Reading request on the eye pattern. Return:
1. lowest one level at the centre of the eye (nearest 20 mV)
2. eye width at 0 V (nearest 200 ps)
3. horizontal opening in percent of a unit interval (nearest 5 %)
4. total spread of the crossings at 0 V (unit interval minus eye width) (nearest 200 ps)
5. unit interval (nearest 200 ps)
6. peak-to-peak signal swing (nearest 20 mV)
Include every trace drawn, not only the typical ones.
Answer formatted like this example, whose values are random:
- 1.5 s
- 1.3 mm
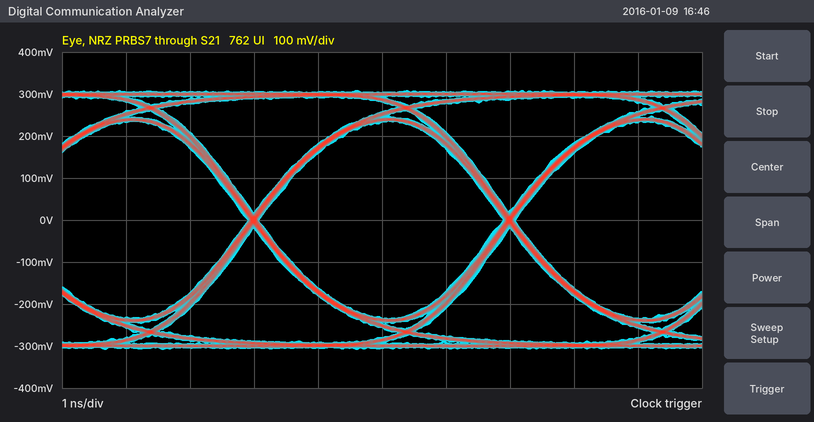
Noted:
- 240 mV
- 3.8 ns
- 95 %
- 200 ps
- 4.0 ns
- 620 mV
